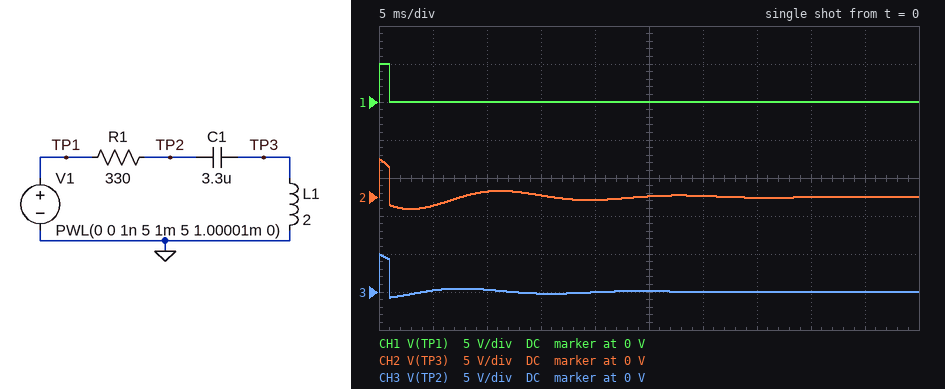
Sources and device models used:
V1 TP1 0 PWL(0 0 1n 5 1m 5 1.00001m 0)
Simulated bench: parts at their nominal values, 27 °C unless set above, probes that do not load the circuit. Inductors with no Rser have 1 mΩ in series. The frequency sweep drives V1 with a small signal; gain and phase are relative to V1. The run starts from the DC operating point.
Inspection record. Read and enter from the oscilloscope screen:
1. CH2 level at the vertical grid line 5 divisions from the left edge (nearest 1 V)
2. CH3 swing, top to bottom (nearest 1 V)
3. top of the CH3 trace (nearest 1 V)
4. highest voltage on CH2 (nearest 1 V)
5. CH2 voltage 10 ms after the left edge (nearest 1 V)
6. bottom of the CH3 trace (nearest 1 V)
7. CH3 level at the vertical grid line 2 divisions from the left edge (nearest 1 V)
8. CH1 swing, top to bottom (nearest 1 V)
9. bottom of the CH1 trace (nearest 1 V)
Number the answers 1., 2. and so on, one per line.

1. 0 V
2. 6 V
3. 5 V
4. 5 V
5. 1 V
6. -1 V
7. 0 V
8. 5 V
9. 0 V
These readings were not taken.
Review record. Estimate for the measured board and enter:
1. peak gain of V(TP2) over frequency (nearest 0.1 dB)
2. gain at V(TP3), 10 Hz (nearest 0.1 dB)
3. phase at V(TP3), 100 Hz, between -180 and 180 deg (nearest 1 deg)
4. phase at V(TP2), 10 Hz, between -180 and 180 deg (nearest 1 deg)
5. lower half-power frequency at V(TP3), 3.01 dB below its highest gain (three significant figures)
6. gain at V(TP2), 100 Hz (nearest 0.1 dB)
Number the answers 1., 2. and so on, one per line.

1. 0 dB
2. -31.5 dB
3. 23 deg
4. -4 deg
5. 53.8 Hz
6. -0.7 dB
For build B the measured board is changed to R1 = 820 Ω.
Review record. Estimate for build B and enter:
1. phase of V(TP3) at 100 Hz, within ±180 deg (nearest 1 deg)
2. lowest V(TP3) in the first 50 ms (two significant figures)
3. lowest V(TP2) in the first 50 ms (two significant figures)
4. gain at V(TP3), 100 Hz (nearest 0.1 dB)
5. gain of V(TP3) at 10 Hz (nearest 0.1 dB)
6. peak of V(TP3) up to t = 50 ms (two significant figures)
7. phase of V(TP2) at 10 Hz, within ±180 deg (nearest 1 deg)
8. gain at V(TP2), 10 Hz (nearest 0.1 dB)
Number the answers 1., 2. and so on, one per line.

1. 47 deg
2. -2.0 V
3. -1.6 V
4. 0.9 dB
5. -31.6 dB
6. 5.0 V
7. -10 deg
8. -0.1 dB
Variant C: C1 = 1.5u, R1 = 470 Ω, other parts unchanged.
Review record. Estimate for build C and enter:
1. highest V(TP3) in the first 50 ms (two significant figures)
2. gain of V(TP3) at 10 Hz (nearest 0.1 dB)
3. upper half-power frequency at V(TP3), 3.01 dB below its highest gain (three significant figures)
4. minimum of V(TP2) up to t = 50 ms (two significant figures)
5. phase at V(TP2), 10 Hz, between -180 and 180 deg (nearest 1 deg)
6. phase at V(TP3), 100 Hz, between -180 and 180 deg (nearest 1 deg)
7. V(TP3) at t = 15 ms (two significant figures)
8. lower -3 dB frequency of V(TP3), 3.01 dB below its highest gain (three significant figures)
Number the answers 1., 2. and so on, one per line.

1. 5.0 V
2. -38.4 dB
3. 128 Hz
4. -990 mV
5. -3 deg
6. 67 deg
7. -390 mV
8. 80.1 Hz
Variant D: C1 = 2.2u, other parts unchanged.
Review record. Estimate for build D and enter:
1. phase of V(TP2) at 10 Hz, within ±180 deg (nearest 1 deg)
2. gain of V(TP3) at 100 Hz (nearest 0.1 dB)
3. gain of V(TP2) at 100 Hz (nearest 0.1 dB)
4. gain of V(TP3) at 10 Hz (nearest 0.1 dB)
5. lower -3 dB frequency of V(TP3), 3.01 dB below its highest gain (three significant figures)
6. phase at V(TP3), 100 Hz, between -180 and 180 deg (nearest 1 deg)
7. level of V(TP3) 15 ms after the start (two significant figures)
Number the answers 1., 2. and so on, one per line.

1. -3 deg
2. 6.0 dB
3. -1.4 dB
4. -35.1 dB
5. 67.0 Hz
6. 32 deg
7. -550 mV
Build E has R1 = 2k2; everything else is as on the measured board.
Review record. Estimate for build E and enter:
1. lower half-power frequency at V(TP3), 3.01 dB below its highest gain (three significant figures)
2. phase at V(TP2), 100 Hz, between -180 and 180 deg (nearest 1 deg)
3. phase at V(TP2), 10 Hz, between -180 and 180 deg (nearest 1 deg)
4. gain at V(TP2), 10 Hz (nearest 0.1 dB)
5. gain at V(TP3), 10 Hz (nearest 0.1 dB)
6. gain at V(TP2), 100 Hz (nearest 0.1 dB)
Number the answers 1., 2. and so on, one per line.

1. 154 Hz
2. 71 deg
3. -25 deg
4. -0.9 dB
5. -32.3 dB
6. -9.6 dB
